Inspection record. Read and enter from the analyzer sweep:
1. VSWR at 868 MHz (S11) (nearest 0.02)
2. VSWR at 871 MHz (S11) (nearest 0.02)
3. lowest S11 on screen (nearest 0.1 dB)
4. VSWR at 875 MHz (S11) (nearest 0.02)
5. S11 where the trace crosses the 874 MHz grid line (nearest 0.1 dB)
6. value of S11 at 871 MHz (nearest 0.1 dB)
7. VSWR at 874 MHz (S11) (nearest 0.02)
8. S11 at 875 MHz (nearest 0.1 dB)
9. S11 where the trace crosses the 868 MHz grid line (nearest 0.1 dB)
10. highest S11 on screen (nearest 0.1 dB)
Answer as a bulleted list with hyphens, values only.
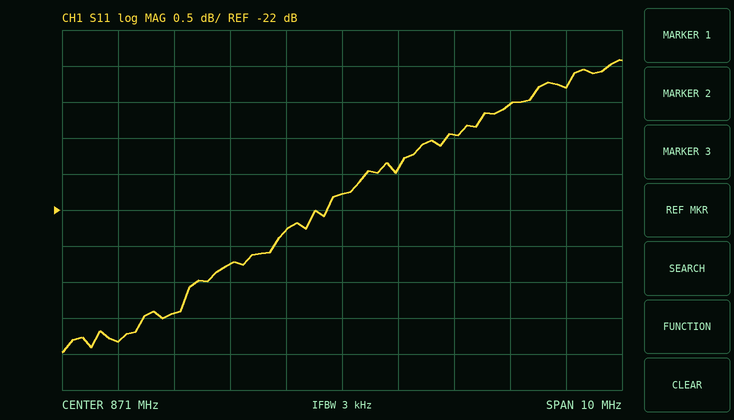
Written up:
- 1.14
- 1.18
- -24.0 dB
- 1.22
- -20.5 dB
- -21.8 dB
- 1.20
- -20.3 dB
- -23.4 dB
- -19.9 dB
